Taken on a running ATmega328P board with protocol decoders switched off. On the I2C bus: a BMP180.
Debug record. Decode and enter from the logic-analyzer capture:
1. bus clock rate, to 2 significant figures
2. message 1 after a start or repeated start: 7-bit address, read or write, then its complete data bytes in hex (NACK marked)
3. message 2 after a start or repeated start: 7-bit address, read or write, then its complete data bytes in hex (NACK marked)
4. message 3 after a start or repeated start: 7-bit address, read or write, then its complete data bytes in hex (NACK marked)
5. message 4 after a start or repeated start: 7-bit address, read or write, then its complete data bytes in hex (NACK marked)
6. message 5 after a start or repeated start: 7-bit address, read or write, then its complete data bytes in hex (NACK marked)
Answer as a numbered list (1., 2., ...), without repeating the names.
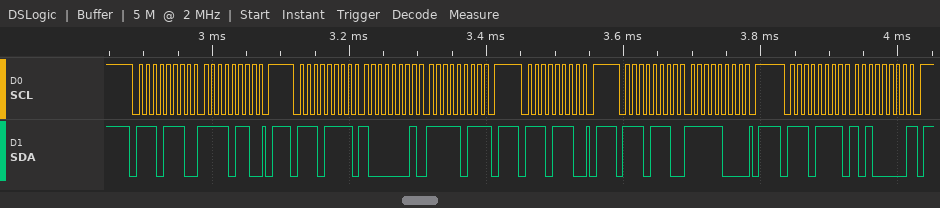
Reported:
1. 100 kHz
2. 0x77 write: F6
3. 0x77 read: 81 FB NACK
4. 0x77 write
5. 0x77 write: F8
6. 0x77 read: A0 NACK
